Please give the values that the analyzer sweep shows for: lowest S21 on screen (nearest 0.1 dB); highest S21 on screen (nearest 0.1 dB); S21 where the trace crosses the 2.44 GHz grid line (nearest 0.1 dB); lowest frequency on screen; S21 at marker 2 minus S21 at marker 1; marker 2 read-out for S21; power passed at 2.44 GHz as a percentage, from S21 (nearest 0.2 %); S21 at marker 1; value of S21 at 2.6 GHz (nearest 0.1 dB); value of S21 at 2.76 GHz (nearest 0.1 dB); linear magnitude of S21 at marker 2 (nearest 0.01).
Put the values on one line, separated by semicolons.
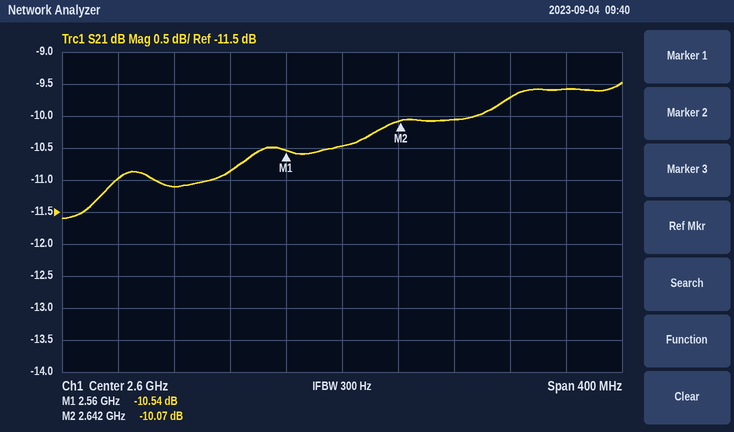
-11.6 dB; -9.5 dB; -11.0 dB; 2.4 GHz; 0.47 dB; -10.07 dB; 8.0 %; -10.54 dB; -10.5 dB; -9.6 dB; 0.31
